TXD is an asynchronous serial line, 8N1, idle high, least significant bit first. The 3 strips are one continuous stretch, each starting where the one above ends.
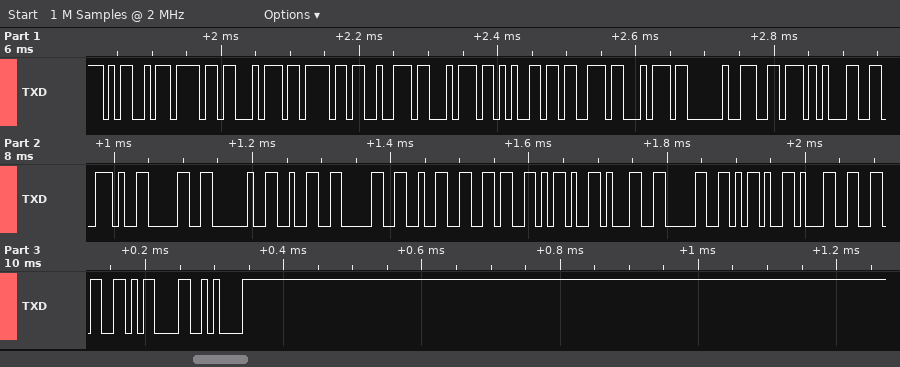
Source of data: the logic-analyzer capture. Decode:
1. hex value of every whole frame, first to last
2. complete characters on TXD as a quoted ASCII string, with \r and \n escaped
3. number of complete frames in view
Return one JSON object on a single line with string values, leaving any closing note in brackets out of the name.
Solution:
{"hex value of every whole frame, first to last": "4D 6F 74 6F 72 74 65 73 74 20 76 31 2E 30 20 32 30 32 36 2D 31 30 2D 31 36 0D 0A", "complete characters on TXD as a quoted ASCII string, with \\r and \\n escaped": "\"Motortest v1.0 2026-10-16\\r\\n\"", "number of complete frames in view": "27"}
